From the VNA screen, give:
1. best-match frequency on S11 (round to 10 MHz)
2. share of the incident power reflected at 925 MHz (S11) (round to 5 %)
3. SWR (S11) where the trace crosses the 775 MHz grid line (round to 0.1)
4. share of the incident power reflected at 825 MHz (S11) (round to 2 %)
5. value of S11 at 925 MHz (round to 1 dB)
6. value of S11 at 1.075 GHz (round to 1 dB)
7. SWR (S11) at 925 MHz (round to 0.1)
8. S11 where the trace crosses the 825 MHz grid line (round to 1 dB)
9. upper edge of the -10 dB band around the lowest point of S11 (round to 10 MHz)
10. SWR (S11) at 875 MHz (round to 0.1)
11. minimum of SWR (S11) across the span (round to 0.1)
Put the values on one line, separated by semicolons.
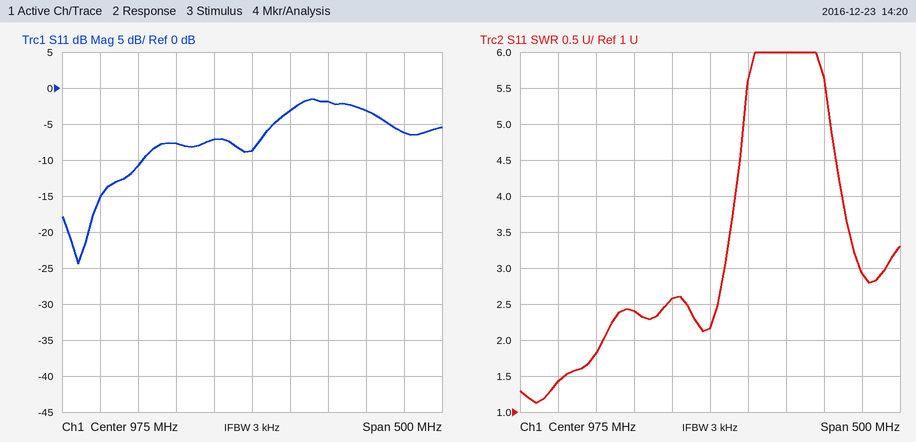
750 MHz; 20 %; 1.4; 8 %; -7 dB; -2 dB; 2.6; -11 dB; 830 MHz; 2.4; 1.1
